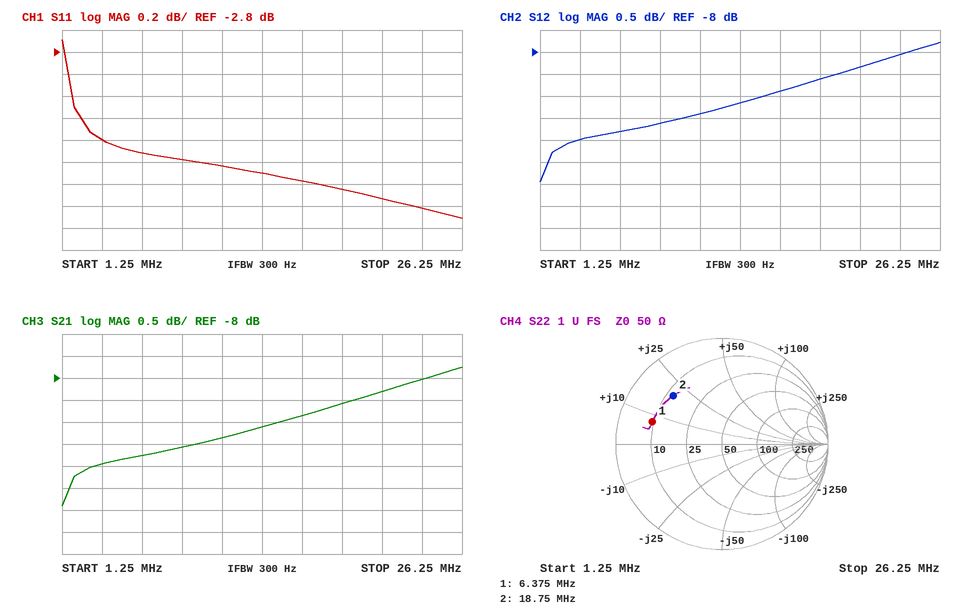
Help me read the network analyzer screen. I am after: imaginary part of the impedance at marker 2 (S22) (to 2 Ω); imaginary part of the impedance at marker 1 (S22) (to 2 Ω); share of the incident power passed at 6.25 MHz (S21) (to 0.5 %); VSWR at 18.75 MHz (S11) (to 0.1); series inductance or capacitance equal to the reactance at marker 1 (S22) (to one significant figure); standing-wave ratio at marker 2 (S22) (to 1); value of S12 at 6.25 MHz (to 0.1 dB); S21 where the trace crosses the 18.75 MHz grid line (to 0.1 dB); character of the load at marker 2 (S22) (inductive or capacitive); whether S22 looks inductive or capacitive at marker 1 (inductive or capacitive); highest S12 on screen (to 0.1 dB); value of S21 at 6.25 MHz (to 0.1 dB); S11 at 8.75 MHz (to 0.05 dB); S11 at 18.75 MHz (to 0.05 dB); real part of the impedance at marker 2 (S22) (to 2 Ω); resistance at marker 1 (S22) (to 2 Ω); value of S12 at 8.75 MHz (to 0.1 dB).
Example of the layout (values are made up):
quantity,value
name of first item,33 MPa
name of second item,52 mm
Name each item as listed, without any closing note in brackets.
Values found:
quantity,value
imaginary part of the impedance at marker 2 (S22),+20 Ω
imaginary part of the impedance at marker 1 (S22),+8 Ω
share of the incident power passed at 6.25 MHz (S21),10.5 %
VSWR at 18.75 MHz (S11),4.4
series inductance or capacitance equal to the reactance at marker 1 (S22),200 nH
standing-wave ratio at marker 2 (S22),5
value of S12 at 6.25 MHz,-9.8 dB
S21 where the trace crosses the 18.75 MHz grid line,-8.6 dB
character of the load at marker 2 (S22),inductive
whether S22 looks inductive or capacitive at marker 1,inductive
highest S12 on screen,-7.8 dB
value of S21 at 6.25 MHz,-9.8 dB
S11 at 8.75 MHz,-3.80 dB
S11 at 18.75 MHz,-4.05 dB
real part of the impedance at marker 2 (S22),12 Ω
resistance at marker 1 (S22),10 Ω
value of S12 at 8.75 MHz,-9.6 dB
